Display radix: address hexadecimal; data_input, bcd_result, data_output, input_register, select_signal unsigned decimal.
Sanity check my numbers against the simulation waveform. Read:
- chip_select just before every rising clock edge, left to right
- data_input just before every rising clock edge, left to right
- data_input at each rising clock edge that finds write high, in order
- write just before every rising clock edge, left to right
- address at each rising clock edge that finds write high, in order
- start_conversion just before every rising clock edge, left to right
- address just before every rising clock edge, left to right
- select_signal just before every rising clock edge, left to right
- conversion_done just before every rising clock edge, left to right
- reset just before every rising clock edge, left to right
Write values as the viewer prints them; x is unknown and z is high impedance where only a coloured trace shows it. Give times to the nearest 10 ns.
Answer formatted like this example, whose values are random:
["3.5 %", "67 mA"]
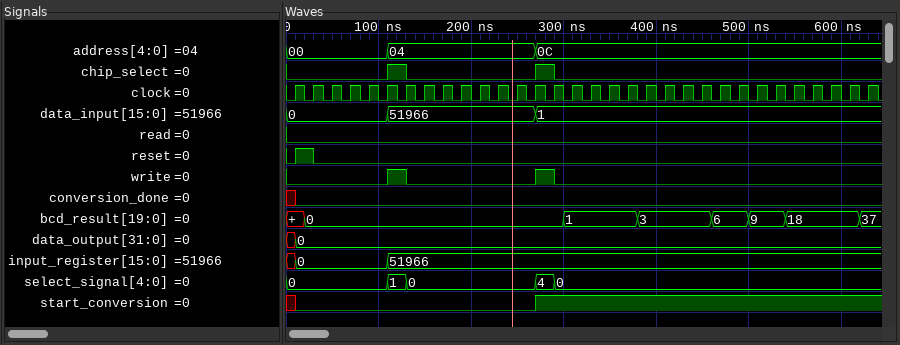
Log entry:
["0 0 0 0 0 0 1 0 0 0 0 0 0 0 1 0 0 0 0 0 0 0 0 0 0 0 0 0 0 0 0 0", "0, 0, 0, 0, 0, 0, 51966, 51966, 51966, 51966, 51966, 51966, 51966, 51966, 1, 1, 1, 1, 1, 1, 1, 1, 1, 1, 1, 1, 1, 1, 1, 1, 1, 1", "51966, 1", "0 0 0 0 0 0 1 0 0 0 0 0 0 0 1 0 0 0 0 0 0 0 0 0 0 0 0 0 0 0 0 0", "04, 0C", "x 0 0 0 0 0 0 0 0 0 0 0 0 0 1 1 1 1 1 1 1 1 1 1 1 1 1 1 1 1 1 1", "00, 00, 00, 00, 00, 00, 04, 04, 04, 04, 04, 04, 04, 04, 0C, 0C, 0C, 0C, 0C, 0C, 0C, 0C, 0C, 0C, 0C, 0C, 0C, 0C, 0C, 0C, 0C, 0C", "0, 0, 0, 0, 0, 0, 1, 0, 0, 0, 0, 0, 0, 0, 4, 0, 0, 0, 0, 0, 0, 0, 0, 0, 0, 0, 0, 0, 0, 0, 0, 0", "x 0 0 0 0 0 0 0 0 0 0 0 0 0 0 0 0 0 0 0 0 0 0 0 0 0 0 0 0 0 0 0", "0 1 0 0 0 0 0 0 0 0 0 0 0 0 0 0 0 0 0 0 0 0 0 0 0 0 0 0 0 0 0 0"]
